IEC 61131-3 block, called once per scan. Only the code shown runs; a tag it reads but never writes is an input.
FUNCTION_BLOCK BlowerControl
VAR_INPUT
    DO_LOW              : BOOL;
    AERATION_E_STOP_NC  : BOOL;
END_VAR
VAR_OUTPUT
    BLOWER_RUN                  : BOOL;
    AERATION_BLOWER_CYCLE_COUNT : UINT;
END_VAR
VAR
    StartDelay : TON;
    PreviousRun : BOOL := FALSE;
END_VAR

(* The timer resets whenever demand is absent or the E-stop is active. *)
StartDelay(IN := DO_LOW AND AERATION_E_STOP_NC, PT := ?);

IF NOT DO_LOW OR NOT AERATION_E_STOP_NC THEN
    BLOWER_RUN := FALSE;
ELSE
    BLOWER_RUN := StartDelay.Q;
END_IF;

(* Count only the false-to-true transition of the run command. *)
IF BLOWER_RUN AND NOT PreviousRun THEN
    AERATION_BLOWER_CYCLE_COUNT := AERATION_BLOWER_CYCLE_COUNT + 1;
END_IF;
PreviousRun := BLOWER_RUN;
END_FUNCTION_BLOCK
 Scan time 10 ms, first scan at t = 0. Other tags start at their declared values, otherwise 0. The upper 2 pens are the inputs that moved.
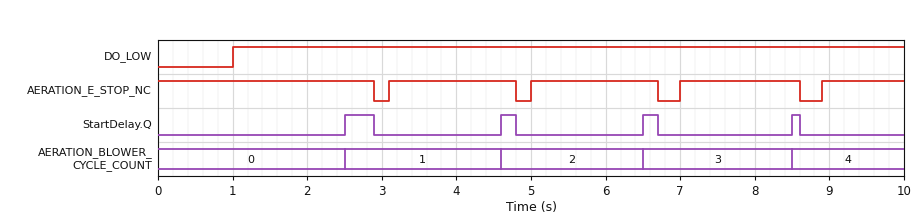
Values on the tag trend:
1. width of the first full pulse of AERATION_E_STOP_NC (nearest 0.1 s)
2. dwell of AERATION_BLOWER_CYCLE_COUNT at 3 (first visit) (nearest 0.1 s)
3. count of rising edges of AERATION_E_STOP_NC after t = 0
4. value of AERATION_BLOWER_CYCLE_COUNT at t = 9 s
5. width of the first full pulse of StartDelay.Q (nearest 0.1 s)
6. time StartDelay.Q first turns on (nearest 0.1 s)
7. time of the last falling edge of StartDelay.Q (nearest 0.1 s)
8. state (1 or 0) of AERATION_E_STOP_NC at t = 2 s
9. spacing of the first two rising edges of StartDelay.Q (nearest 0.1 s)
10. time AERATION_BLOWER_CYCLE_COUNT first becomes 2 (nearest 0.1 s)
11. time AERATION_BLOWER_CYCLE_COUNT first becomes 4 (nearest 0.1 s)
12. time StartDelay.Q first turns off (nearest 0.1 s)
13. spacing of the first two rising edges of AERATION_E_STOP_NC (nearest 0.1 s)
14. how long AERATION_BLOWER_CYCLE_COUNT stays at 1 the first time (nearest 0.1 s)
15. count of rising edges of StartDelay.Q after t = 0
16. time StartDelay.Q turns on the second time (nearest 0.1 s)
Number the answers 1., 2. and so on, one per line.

1. 1.7 s
2. 2.0 s
3. 4
4. 4
5. 0.4 s
6. 2.5 s
7. 8.6 s
8. 1
9. 2.1 s
10. 4.6 s
11. 8.5 s
12. 2.9 s
13. 1.9 s
14. 2.1 s
15. 4
16. 4.6 s
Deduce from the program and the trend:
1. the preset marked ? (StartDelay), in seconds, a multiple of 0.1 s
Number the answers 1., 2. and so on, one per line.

1. 1.5 s
